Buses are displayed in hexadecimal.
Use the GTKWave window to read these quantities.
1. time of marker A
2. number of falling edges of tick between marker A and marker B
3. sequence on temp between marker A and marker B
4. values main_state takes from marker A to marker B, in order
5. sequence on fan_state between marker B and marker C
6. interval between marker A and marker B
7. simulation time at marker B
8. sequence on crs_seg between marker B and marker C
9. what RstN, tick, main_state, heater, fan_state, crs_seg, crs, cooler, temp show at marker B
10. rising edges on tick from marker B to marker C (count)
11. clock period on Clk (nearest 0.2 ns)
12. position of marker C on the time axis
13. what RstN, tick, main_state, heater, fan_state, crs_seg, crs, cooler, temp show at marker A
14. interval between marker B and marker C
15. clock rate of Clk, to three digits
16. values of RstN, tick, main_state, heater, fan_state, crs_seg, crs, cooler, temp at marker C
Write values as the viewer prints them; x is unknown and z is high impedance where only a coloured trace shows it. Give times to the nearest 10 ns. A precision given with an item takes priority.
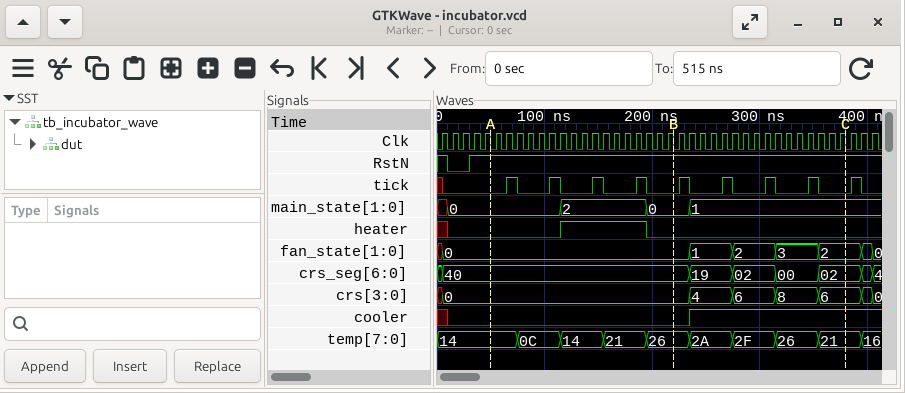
50 ns
4
14, 0C, 14, 21, 26
0, 2, 0
0, 1, 2, 3, 2
170 ns
220 ns
40, 19, 02, 00, 02
RstN=1, tick=0, main_state=0, heater=0, fan_state=0, crs_seg=40, crs=0, cooler=0, temp=26
4
10 ns
380 ns
RstN=1, tick=0, main_state=0, heater=0, fan_state=0, crs_seg=40, crs=0, cooler=0, temp=14
160 ns
100 MHz
RstN=1, tick=0, main_state=1, heater=0, fan_state=2, crs_seg=02, crs=6, cooler=1, temp=21
